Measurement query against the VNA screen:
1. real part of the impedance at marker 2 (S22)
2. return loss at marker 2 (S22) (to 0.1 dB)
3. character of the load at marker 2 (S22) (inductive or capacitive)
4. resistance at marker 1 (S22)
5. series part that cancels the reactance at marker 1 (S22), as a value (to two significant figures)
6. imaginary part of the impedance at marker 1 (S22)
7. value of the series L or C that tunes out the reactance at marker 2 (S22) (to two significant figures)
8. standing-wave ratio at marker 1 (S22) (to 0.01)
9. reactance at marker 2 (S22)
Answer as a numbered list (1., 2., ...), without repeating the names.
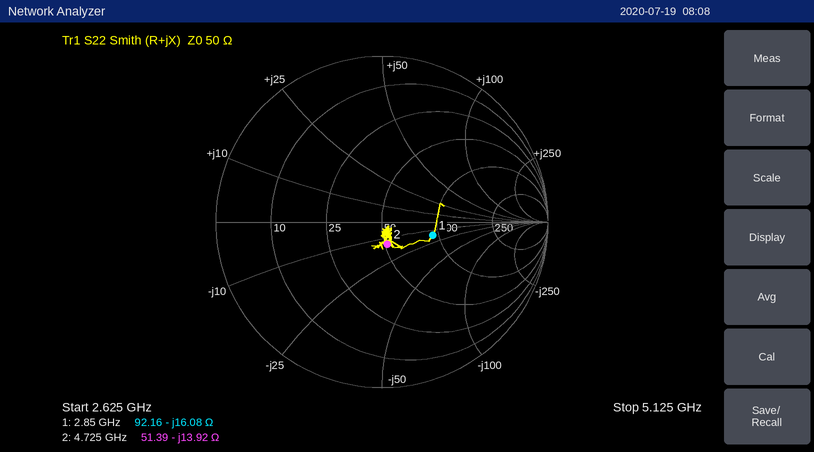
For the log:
1. 51.39 Ω
2. 17.3 dB
3. capacitive
4. 92.16 Ω
5. 900 pH
6. -16.08 Ω
7. 470 pH
8. 1.92
9. -13.92 Ω
